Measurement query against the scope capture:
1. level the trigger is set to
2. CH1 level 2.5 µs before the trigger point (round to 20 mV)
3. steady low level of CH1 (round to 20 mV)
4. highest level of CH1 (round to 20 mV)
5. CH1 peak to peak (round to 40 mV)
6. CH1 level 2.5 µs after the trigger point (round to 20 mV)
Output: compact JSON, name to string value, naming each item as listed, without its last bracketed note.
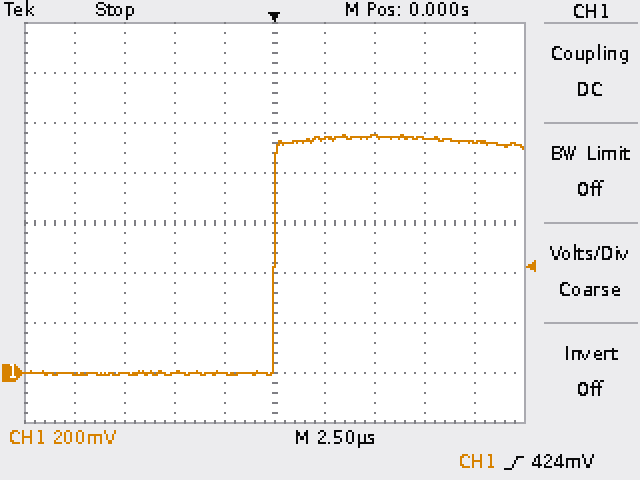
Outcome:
{"level the trigger is set to": "424 mV", "CH1 level 2.5 µs before the trigger point": "0 mV", "steady low level of CH1": "0 mV", "highest level of CH1": "960 mV", "CH1 peak to peak": "960 mV", "CH1 level 2.5 µs after the trigger point": "940 mV"}
